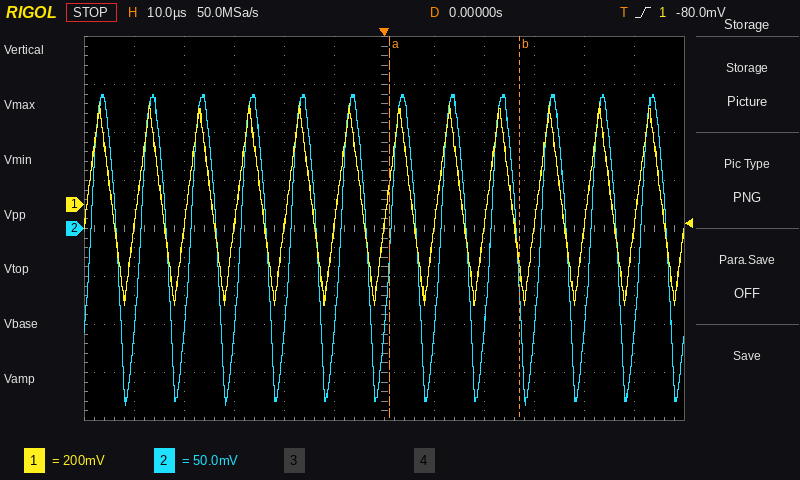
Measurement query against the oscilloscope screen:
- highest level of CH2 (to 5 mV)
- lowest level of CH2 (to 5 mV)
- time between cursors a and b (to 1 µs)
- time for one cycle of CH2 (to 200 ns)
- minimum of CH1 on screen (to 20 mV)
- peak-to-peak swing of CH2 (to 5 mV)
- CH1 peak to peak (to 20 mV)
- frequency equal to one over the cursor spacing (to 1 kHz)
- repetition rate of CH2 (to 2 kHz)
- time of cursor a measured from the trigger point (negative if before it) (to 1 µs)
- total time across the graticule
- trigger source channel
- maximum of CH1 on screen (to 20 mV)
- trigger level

140 mV
-185 mV
26 µs
10.0 µs
-420 mV
325 mV
840 mV
38 kHz
100 kHz
+1 µs
120 µs
CH1
420 mV
-80.0 mV
